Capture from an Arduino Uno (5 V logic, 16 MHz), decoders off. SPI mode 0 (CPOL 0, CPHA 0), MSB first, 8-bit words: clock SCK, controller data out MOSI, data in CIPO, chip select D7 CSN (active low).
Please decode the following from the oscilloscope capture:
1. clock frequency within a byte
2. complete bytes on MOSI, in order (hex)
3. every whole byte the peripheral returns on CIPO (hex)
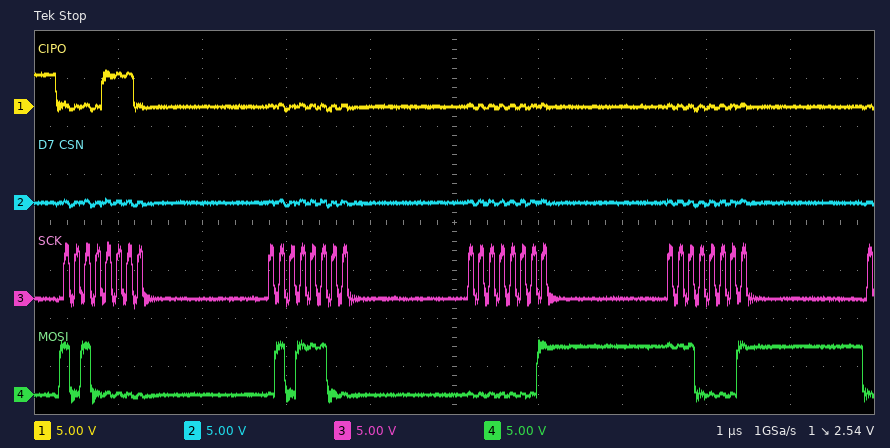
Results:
8 MHz
A0 5C 01 E1
0E 00 00 00
